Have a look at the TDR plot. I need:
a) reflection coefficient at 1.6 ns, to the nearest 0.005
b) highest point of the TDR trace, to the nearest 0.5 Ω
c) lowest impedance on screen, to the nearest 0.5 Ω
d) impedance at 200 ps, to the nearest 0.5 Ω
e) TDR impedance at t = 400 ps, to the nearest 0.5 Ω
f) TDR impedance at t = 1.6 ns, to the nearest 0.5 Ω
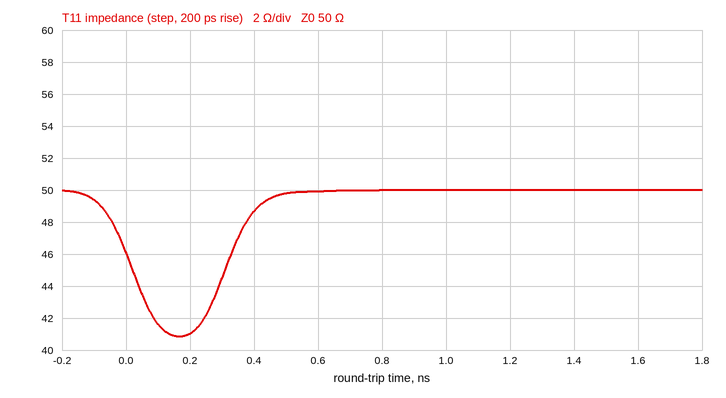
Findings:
0.000
50.0 Ω
41.0 Ω
41.0 Ω
48.5 Ω
50.0 Ω
